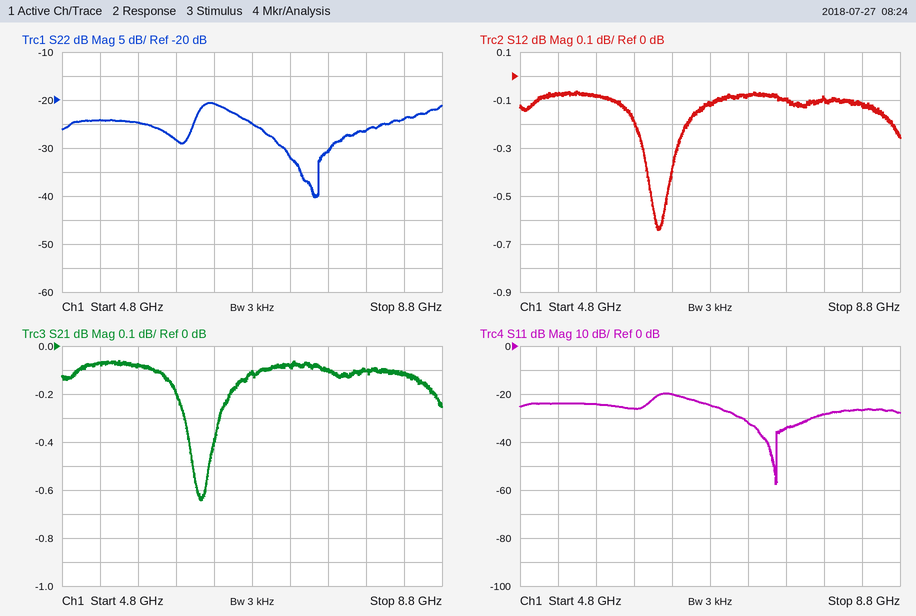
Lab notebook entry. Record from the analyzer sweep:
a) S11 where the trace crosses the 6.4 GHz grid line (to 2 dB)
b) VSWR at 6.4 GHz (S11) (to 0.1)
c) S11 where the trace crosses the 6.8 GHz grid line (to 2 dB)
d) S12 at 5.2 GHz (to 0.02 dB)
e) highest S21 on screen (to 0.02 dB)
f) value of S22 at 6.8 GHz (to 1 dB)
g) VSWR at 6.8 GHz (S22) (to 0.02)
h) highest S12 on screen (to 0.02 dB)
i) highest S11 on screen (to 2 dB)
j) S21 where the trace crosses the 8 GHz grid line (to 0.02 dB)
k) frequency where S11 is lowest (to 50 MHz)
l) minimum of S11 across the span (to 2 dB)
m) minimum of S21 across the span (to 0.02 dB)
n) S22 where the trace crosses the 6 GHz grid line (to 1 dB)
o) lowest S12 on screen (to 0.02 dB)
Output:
-20 dB
1.2
-24 dB
-0.08 dB
-0.06 dB
-25 dB
1.12
-0.06 dB
-20 dB
-0.10 dB
7.50 GHz
-58 dB
-0.64 dB
-28 dB
-0.64 dB
